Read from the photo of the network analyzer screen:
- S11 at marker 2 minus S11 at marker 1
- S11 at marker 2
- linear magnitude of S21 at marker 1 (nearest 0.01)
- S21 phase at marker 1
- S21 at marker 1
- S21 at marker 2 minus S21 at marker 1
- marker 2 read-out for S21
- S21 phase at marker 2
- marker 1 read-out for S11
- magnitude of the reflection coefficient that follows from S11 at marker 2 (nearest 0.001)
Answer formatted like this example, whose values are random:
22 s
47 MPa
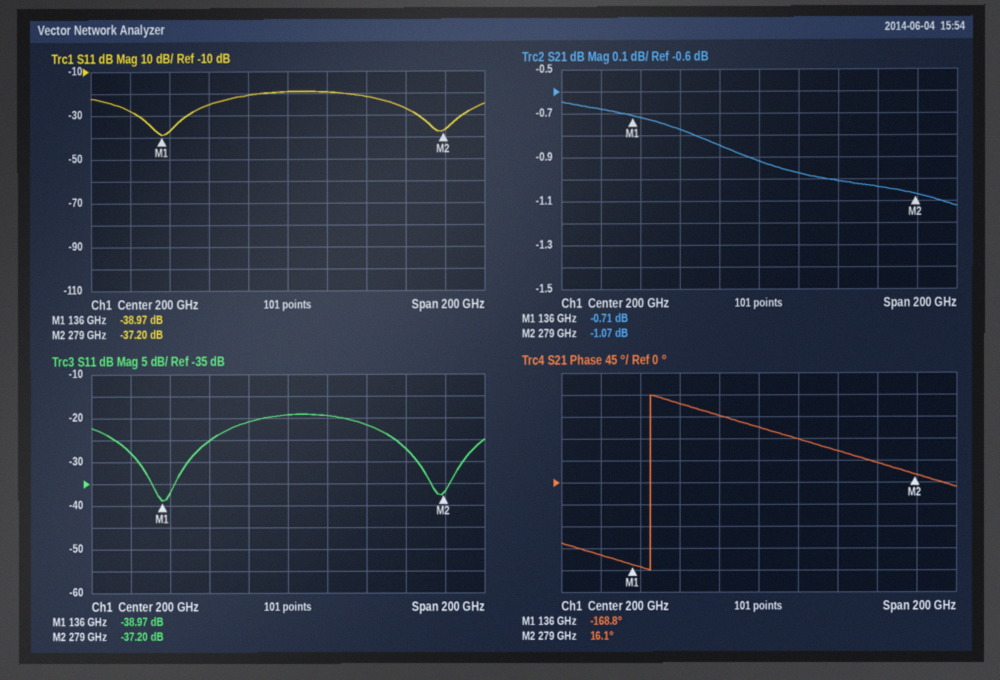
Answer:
1.77 dB
-37.20 dB
0.92
-168.8°
-0.71 dB
-0.36 dB
-1.07 dB
16.1°
-38.97 dB
0.014
